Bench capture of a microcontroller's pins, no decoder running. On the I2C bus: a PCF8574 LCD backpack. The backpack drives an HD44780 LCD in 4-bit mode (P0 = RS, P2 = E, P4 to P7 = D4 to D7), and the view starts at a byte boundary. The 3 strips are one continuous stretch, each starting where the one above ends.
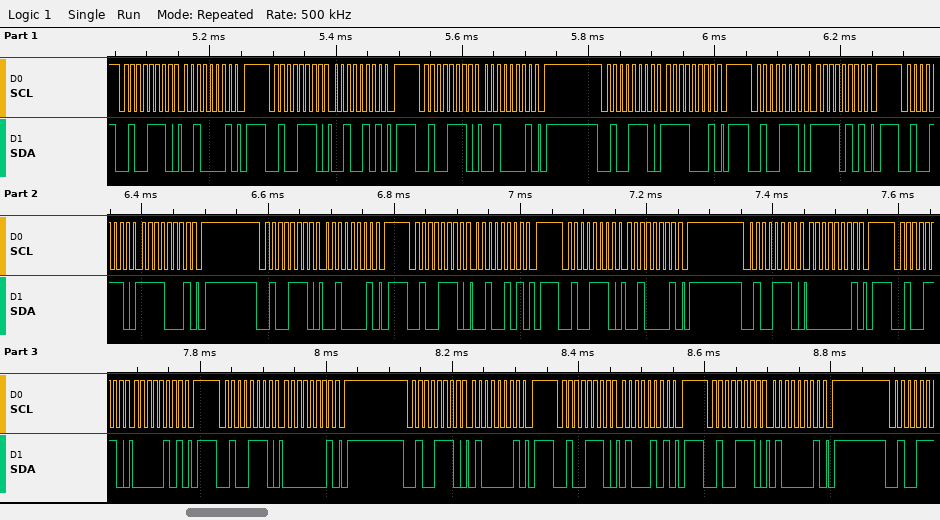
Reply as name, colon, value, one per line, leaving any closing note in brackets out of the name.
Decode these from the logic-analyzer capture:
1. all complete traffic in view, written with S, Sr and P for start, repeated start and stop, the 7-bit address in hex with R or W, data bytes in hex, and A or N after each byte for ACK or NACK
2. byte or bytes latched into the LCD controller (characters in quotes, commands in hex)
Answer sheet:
all complete traffic in view, written with S, Sr and P for start, repeated start and stop, the 7-bit address in hex with R or W, data bytes in hex, and A or N after each byte for ACK or NACK: S 27W A 21 A P S 27W A 25 A P S 27W A 21 A P S 27W A F1 A P S 27W A F5 A P S 27W A F1 A P S 27W A 21 A P S 27W A 25 A P S 27W A 21 A P S 27W A 01 A P S 27W A 05 A P S 27W A 01 A P S 27W A 41 A P S 27W A 45 A P S 27W A 41 A P
byte or bytes latched into the LCD controller: '/' ' '
